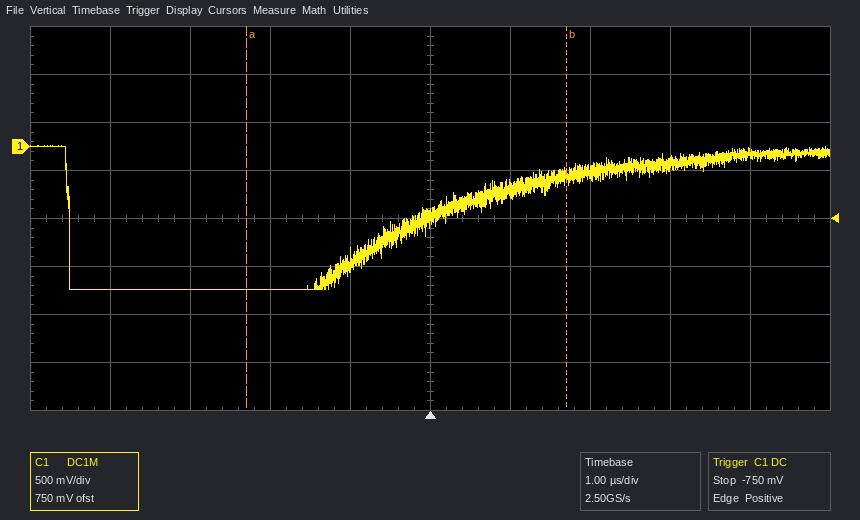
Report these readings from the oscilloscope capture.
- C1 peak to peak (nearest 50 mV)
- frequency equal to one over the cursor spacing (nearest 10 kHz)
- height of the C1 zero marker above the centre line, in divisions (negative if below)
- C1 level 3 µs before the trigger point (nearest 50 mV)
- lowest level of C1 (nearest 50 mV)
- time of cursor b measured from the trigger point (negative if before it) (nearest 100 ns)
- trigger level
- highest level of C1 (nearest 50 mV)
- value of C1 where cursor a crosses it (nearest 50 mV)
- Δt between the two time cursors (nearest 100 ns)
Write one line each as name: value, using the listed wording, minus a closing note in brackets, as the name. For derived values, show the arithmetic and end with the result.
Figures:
C1 peak to peak: 0 mV − (-1.50 V) = 1.50 V
frequency equal to one over the cursor spacing: 1 / 4.0 µs ≈ 250 kHz
height of the C1 zero marker above the centre line, in divisions: +1.5 div
C1 level 3 µs before the trigger point: -1.50 V
lowest level of C1: -1.50 V
time of cursor b measured from the trigger point (negative if before it): +1.7 µs
trigger level: -750 mV
highest level of C1: 0 mV
value of C1 where cursor a crosses it: -1.50 V
Δt between the two time cursors: 4.0 µs
